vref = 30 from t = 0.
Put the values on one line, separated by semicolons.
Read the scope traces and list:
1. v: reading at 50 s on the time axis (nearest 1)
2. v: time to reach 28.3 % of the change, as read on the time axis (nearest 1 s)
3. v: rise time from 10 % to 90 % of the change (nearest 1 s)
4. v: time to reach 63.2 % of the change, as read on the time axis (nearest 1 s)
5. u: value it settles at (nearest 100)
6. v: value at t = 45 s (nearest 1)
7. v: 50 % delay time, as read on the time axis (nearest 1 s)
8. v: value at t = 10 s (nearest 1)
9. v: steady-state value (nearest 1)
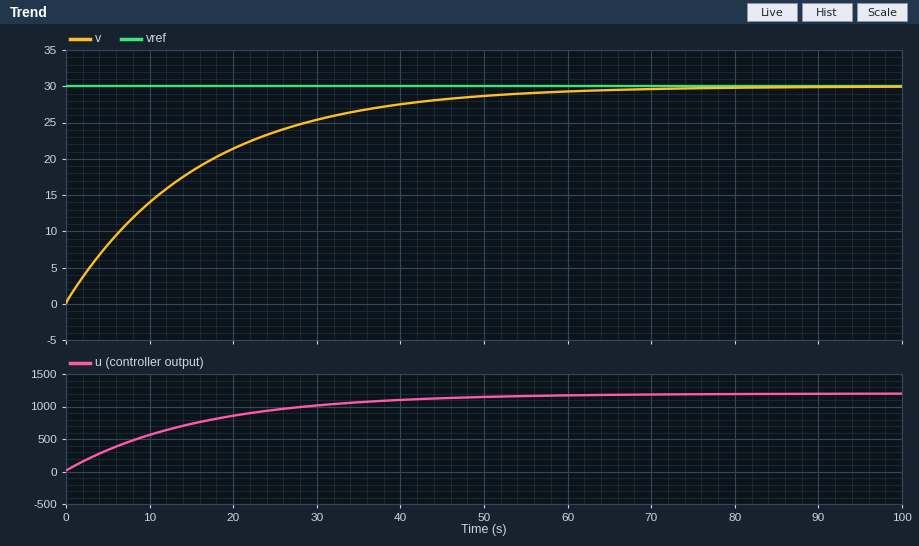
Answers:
29; 5 s; 35 s; 16 s; 1200; 28; 11 s; 14; 30
